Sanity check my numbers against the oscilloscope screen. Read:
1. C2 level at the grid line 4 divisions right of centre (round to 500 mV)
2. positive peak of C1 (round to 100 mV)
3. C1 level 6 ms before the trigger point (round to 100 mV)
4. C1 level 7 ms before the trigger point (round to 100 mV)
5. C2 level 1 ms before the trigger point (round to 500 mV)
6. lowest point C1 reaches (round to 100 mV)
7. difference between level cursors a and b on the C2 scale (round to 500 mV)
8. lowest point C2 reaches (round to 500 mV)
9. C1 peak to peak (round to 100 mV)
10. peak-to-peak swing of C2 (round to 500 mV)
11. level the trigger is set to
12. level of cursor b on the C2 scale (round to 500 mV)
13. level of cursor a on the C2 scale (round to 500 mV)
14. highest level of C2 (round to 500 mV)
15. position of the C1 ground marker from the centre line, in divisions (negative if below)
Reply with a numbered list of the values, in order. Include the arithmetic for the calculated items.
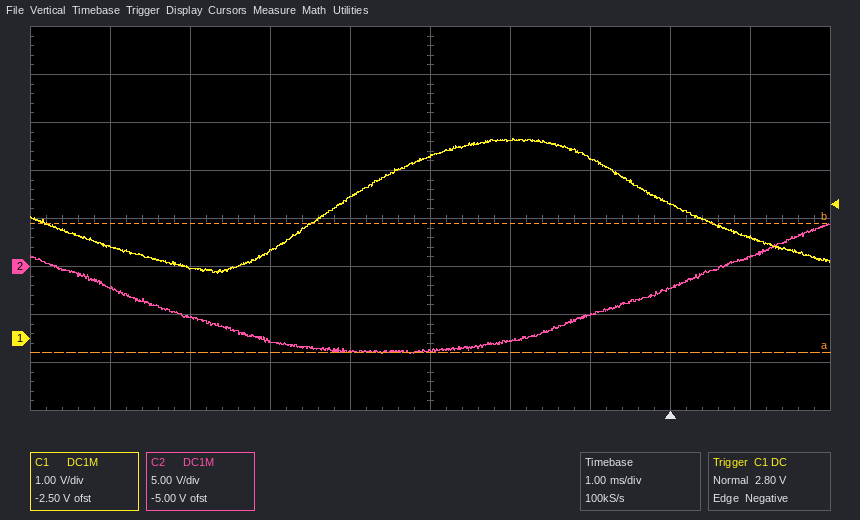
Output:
1. 1.0 V
2. 4.2 V
3. 1.5 V
4. 1.9 V
5. -5.0 V
6. 1.4 V
7. 13.5 V
8. -9.0 V
9. 4.2 V − (1.4 V) = 2.8 V
10. 4.5 V − (-9.0 V) = 13.5 V
11. 2.80 V
12. 4.5 V
13. -9.0 V
14. 4.5 V
15. -2.5 div
